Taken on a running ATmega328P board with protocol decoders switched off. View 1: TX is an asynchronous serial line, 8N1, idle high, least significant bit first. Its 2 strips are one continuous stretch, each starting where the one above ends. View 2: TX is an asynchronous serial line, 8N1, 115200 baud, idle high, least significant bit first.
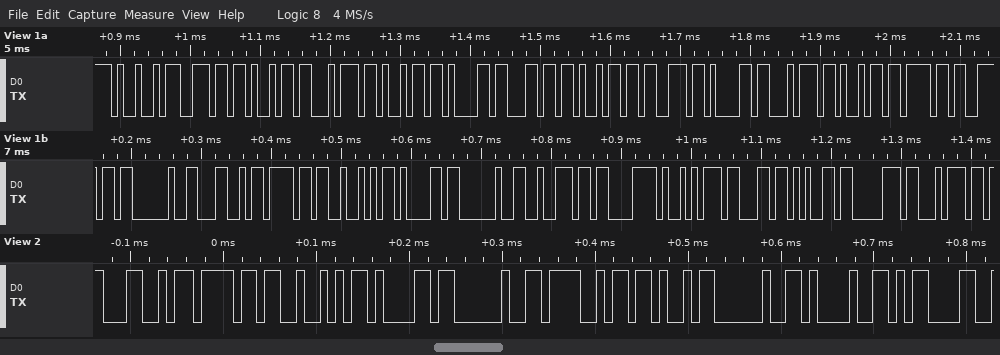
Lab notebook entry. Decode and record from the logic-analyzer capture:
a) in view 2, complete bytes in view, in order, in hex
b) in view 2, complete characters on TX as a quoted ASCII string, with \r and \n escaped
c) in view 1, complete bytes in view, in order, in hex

4C 6F 52 61 20 4F 4B 20 21 0D
"LoRa OK !\r"
49 6E 69 74 69 61 6C 69 73 61 74 69 6F 6E 20 4C 6F 52 61 20 72 C3 A9 63 65 70 74
